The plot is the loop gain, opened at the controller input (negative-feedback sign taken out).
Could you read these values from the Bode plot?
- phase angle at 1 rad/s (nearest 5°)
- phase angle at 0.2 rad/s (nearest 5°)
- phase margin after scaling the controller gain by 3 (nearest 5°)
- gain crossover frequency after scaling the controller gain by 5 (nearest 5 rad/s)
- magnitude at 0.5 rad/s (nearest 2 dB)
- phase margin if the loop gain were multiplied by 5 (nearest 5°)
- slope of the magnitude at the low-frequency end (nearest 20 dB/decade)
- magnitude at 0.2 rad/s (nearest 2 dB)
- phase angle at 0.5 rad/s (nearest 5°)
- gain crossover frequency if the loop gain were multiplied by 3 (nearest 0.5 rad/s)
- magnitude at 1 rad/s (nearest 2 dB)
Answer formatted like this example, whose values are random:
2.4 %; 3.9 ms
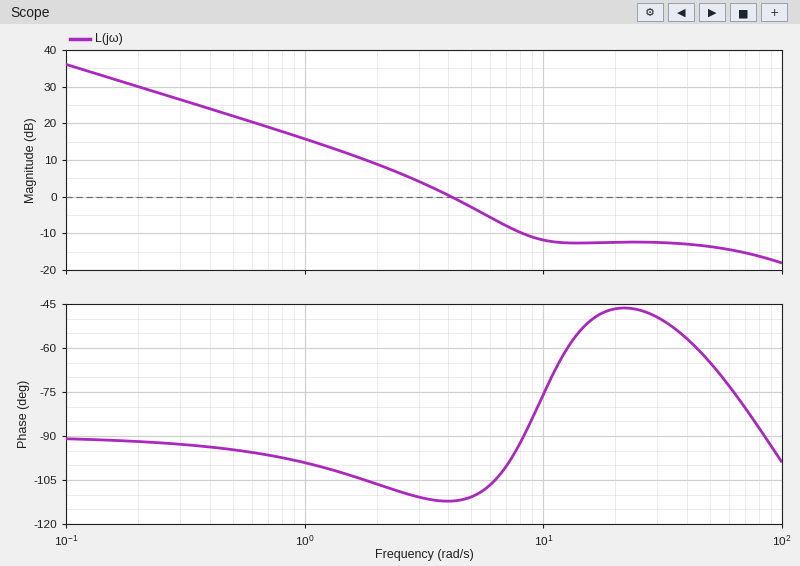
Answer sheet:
-100°; -90°; 85°; 55 rad/s; 22 dB; 110°; -20 dB/decade; 30 dB; -95°; 8.0 rad/s; 16 dB
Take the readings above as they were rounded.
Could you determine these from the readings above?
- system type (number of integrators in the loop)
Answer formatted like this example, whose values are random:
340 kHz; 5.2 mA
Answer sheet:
1
